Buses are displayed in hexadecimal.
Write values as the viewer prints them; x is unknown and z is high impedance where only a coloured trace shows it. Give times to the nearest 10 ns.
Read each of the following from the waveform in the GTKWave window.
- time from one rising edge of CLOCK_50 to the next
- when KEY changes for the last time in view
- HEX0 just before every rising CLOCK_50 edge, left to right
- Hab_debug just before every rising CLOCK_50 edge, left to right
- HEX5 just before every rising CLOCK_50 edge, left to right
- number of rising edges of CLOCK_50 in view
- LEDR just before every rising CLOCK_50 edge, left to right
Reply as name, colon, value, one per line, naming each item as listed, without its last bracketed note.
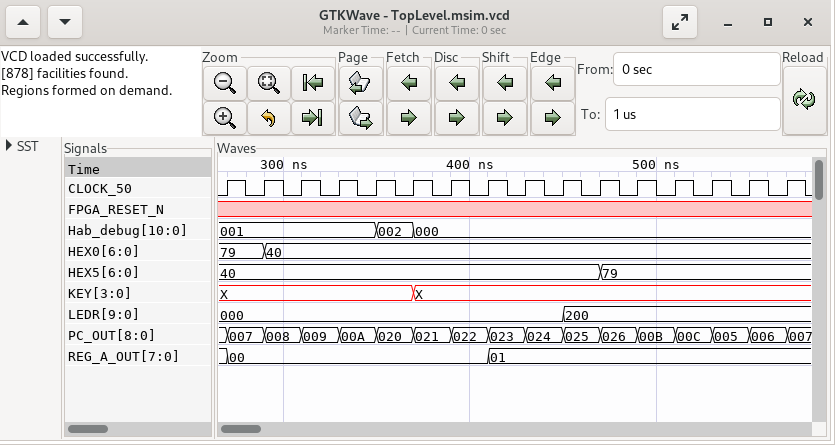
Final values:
time from one rising edge of CLOCK_50 to the next: 20 ns
when KEY changes for the last time in view: 370 ns
HEX0 just before every rising CLOCK_50 edge, left to right: 79, 79, 40, 40, 40, 40, 40, 40, 40, 40, 40, 40, 40, 40, 40, 40
Hab_debug just before every rising CLOCK_50 edge, left to right: 001, 001, 001, 001, 001, 002, 000, 000, 000, 000, 000, 000, 000, 000, 000, 000
HEX5 just before every rising CLOCK_50 edge, left to right: 40, 40, 40, 40, 40, 40, 40, 40, 40, 40, 40, 79, 79, 79, 79, 79
number of rising edges of CLOCK_50 in view: 16
LEDR just before every rising CLOCK_50 edge, left to right: 000, 000, 000, 000, 000, 000, 000, 000, 000, 000, 200, 200, 200, 200, 200, 200
